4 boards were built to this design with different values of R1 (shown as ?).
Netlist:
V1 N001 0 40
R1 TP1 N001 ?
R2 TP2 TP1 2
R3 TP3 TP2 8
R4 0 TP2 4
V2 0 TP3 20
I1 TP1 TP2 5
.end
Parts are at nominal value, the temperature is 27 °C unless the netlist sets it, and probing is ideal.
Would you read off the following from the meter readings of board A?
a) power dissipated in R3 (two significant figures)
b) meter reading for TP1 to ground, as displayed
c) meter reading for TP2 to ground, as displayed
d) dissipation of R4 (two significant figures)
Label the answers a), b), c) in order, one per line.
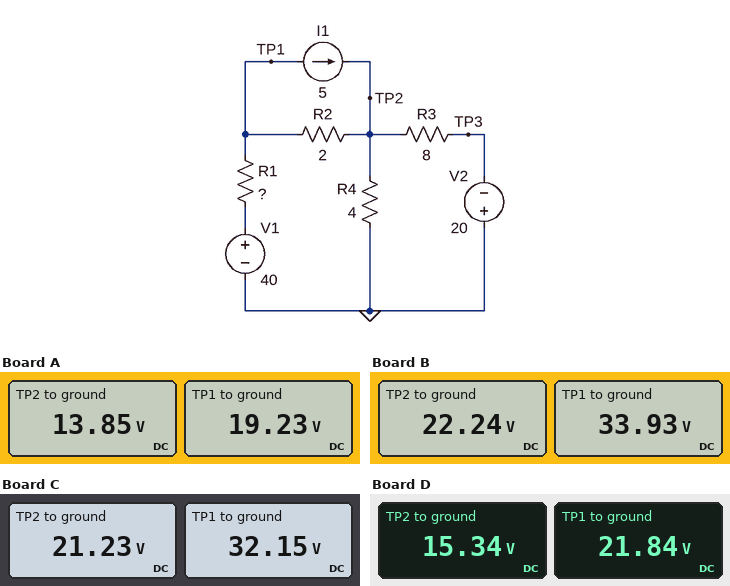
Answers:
a) 140 W
b) 19.23 V
c) 13.85 V
d) 48 W
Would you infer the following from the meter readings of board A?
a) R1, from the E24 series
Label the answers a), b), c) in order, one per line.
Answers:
a) 2.7 Ω
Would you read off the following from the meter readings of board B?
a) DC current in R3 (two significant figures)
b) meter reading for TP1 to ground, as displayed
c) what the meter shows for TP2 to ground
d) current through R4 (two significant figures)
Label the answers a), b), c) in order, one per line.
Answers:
a) 5.3 A
b) 33.93 V
c) 22.24 V
d) 5.6 A
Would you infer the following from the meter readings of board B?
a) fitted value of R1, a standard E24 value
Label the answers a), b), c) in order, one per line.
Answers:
a) 0.56 Ω
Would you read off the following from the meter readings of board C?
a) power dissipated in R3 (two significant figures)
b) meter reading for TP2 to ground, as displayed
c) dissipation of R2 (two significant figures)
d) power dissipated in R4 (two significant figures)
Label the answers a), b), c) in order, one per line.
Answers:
a) 210 W
b) 21.23 V
c) 60 W
d) 110 W
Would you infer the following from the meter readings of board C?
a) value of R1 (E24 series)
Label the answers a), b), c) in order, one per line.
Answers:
a) 0.75 Ω
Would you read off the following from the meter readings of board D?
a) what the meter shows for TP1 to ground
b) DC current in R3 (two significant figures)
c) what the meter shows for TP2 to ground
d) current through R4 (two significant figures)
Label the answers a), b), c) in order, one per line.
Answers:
a) 21.84 V
b) 4.4 A
c) 15.34 V
d) 3.8 A
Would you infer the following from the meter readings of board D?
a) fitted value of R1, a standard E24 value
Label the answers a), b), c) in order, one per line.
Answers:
a) 2.2 Ω
